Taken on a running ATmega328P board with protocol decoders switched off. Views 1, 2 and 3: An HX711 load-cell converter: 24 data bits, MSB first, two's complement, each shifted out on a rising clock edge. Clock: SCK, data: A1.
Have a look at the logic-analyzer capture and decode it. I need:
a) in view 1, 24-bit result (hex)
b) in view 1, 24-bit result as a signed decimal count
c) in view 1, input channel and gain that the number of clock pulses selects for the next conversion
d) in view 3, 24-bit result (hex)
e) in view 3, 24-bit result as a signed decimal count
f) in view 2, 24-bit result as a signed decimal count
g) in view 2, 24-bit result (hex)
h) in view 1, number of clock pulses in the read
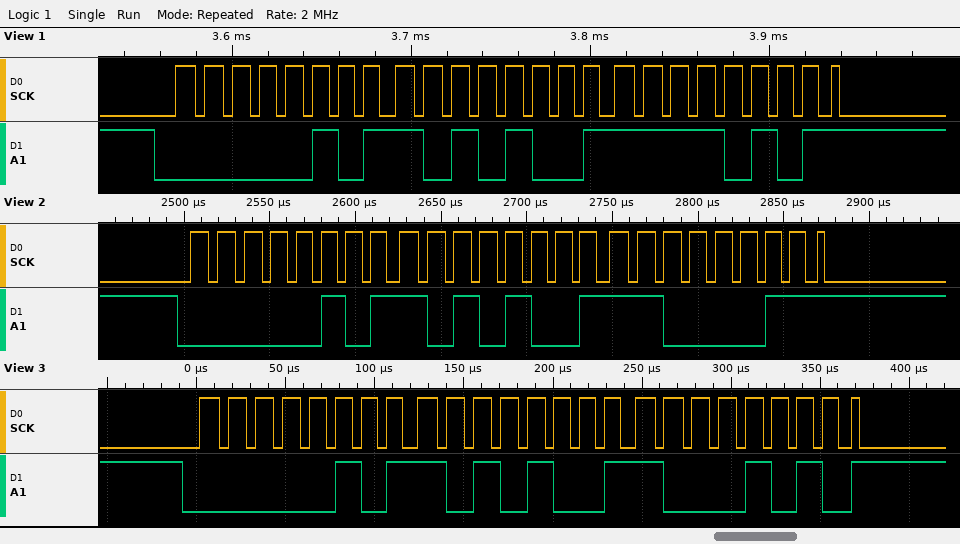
0x05A9F5
371189
channel A, gain 128
0x05A98A
371082
371139
0x05A9C3
25
